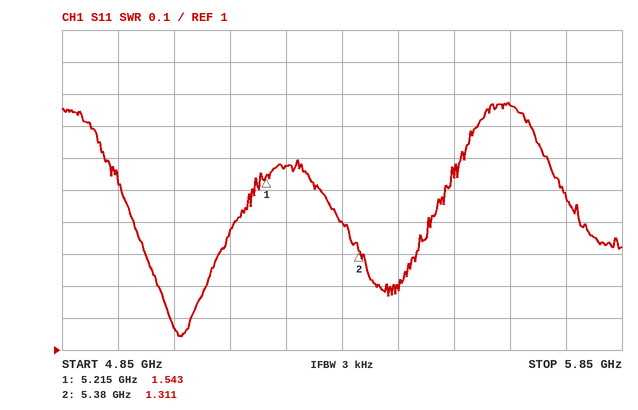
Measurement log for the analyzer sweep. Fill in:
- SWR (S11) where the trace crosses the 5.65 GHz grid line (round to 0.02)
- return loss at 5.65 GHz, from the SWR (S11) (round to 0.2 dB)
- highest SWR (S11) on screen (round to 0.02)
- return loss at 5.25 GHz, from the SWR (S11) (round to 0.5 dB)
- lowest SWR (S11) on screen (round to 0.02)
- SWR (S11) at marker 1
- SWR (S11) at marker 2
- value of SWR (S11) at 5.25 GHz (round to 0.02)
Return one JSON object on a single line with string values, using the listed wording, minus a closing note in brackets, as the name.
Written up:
{"SWR (S11) where the trace crosses the 5.65 GHz grid line": "1.76", "return loss at 5.65 GHz, from the SWR (S11)": "11.2 dB", "highest SWR (S11) on screen": "1.78", "return loss at 5.25 GHz, from the SWR (S11)": "13.0 dB", "lowest SWR (S11) on screen": "1.04", "SWR (S11) at marker 1": "1.543", "SWR (S11) at marker 2": "1.311", "value of SWR (S11) at 5.25 GHz": "1.58"}
